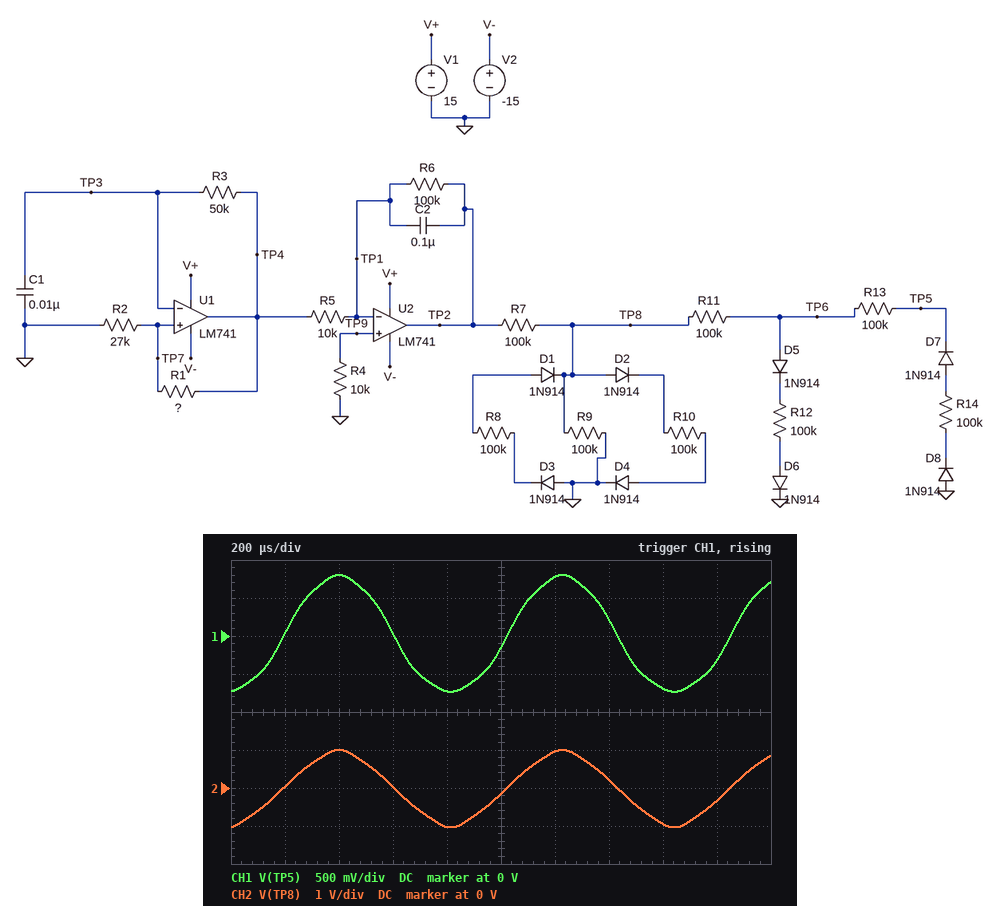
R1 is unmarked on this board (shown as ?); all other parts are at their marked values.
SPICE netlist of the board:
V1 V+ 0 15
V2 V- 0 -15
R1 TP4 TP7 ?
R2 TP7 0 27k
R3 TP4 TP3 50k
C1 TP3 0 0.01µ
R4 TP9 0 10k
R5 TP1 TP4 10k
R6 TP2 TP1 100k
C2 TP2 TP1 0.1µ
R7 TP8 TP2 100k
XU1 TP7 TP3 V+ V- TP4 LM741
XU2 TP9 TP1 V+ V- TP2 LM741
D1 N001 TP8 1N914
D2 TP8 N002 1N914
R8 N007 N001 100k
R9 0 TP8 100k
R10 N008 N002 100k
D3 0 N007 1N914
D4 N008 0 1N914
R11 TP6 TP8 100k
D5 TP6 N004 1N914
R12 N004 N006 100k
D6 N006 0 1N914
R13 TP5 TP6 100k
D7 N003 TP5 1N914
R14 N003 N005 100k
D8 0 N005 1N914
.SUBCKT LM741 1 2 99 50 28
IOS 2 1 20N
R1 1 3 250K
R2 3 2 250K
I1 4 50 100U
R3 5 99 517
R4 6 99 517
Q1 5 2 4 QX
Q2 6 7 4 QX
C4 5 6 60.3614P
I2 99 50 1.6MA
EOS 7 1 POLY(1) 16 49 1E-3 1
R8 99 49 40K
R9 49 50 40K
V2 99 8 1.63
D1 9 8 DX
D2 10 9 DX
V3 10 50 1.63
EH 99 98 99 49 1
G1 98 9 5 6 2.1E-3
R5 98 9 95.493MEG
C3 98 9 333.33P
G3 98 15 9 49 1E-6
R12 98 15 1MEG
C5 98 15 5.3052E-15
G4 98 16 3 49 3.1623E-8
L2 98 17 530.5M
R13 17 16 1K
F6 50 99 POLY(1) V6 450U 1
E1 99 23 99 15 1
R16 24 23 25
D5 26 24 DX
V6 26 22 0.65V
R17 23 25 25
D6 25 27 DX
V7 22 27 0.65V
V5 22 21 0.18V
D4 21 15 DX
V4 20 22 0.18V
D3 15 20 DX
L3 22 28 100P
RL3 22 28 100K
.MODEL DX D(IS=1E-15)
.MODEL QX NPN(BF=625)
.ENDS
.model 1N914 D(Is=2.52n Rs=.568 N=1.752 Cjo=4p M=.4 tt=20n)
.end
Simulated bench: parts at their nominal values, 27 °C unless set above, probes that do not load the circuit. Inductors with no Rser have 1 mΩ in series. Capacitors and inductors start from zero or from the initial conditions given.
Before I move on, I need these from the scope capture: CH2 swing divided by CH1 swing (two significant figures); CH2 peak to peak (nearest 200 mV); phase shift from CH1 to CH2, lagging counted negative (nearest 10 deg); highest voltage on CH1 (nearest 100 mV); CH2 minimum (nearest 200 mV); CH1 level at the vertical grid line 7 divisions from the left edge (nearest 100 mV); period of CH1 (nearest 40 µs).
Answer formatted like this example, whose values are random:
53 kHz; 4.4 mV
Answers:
1.3; 2.0 V; 0 deg; 800 mV; -1.0 V; 200 mV; 840 µs
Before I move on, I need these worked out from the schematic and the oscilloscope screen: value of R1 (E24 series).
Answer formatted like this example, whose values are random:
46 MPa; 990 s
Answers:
51 kΩ
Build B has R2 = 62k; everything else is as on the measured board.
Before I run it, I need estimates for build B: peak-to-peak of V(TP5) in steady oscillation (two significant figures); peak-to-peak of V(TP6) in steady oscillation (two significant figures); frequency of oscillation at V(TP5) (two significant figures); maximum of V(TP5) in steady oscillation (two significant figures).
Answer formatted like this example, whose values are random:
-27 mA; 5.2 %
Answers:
2.0 V; 2.3 V; 770 Hz; 1.1 V
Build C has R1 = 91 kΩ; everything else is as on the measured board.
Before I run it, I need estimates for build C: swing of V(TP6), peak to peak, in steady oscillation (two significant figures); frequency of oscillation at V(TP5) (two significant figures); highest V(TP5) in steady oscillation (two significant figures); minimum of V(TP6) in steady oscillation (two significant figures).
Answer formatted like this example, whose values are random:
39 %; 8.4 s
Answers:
1.3 V; 1.7 kHz; 640 mV; -690 mV
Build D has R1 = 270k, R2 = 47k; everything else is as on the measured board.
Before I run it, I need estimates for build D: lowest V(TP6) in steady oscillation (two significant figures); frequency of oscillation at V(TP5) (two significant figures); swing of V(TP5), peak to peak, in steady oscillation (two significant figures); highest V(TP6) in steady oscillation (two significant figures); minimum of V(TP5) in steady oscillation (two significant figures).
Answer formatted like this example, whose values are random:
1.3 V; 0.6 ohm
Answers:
-540 mV; 2.3 kHz; 1.0 V; 510 mV; -500 mV
